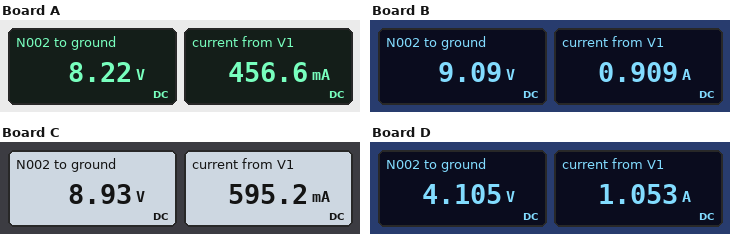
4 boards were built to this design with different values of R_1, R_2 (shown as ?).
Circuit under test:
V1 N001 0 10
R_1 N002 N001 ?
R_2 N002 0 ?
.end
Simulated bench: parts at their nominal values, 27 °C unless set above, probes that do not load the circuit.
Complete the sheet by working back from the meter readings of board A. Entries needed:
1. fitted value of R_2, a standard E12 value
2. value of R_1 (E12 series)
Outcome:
18 Ω
3.9 Ω
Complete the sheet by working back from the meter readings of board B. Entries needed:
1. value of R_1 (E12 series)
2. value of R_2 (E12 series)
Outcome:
1 Ω
10 Ω
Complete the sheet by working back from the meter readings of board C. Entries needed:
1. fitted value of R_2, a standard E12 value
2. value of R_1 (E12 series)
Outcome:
15 Ω
1.8 Ω
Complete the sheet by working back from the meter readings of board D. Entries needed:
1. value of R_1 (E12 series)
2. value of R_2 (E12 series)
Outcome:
5.6 Ω
3.9 Ω
